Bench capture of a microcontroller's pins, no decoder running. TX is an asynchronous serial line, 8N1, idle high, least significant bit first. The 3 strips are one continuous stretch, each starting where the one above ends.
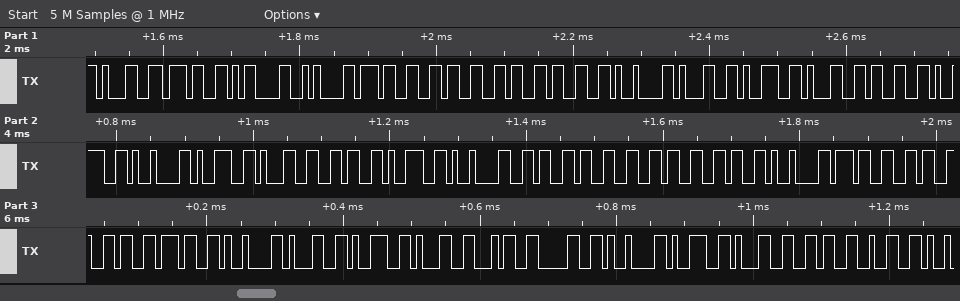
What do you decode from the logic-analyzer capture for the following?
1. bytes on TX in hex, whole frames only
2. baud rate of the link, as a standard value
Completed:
0x31 0x37 0x0D 0x0A 0x37 0x36 0x36 0x33 0x09 0x31 0x39 0x31 0x33 0x39 0x09 0x39 0x31 0x36 0x39 0x09 0x36 0x33 0x36 0x36 0x09 0x37 0x36 0x36 0x37 0x09 0x31 0x39 0x31 0x34 0x30 0x09 0x39 0x31 0x36 0x32
115200 baud
